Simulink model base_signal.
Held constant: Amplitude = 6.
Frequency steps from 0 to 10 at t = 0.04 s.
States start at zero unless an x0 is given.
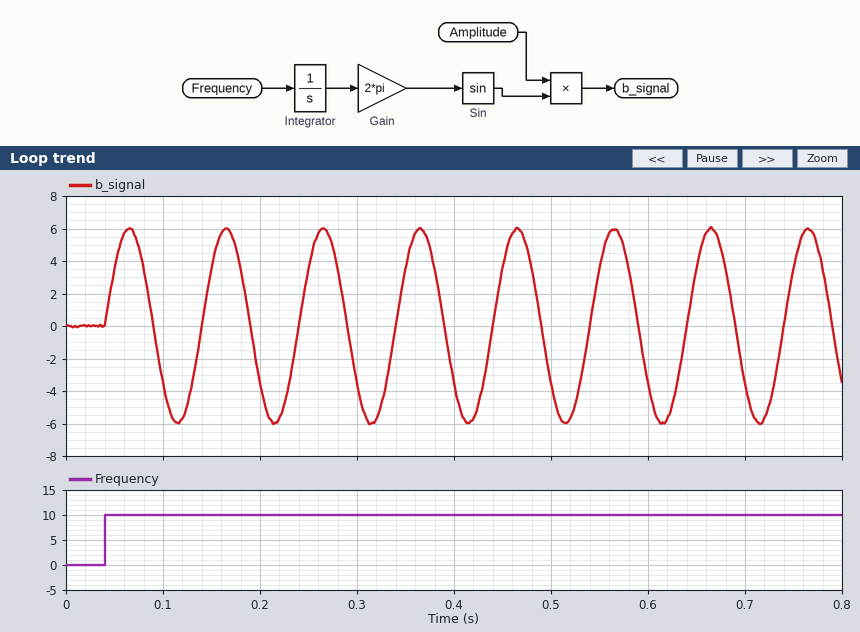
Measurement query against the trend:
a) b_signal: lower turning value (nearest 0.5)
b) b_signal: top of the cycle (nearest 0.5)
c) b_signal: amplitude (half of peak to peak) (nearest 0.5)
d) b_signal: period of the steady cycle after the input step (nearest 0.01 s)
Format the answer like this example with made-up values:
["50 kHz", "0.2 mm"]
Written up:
["-6.0", "6.0", "6.0", "0.10 s"]
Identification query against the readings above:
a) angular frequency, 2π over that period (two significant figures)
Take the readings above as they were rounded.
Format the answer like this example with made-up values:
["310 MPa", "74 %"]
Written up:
["63 rad/s"]
